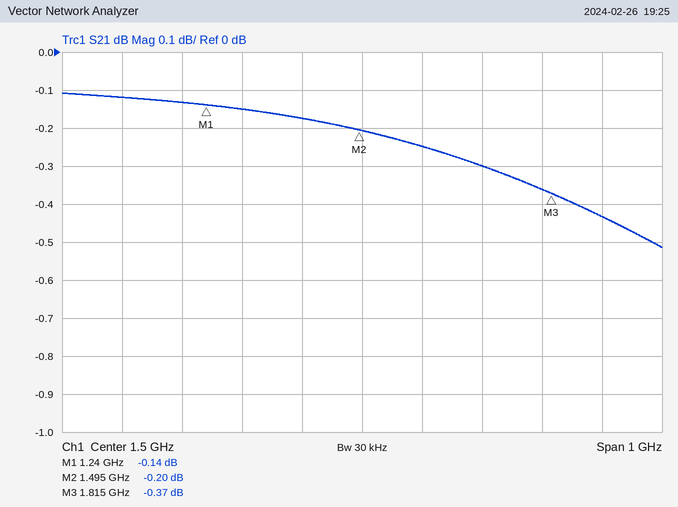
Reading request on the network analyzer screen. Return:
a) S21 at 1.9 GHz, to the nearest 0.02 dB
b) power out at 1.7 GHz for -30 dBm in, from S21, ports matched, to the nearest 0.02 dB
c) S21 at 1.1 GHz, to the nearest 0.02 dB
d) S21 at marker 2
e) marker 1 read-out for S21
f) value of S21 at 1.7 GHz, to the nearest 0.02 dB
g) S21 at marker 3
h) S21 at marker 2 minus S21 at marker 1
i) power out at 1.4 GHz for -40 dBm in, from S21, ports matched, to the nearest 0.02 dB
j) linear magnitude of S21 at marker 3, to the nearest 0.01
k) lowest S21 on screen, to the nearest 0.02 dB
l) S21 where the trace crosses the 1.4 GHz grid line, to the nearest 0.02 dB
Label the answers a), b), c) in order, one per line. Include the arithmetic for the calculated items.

a) -0.44 dB
b) -30 dBm + (-0.30 dB) = -30.30 dBm
c) -0.12 dB
d) -0.20 dB
e) -0.14 dB
f) -0.30 dB
g) -0.37 dB
h) -0.2 − (-0.14) = -0.06 dB
i) -40 dBm + (-0.18 dB) = -40.18 dBm
j) 10^(-0.37/20) ≈ 0.96
k) -0.52 dB
l) -0.18 dB
